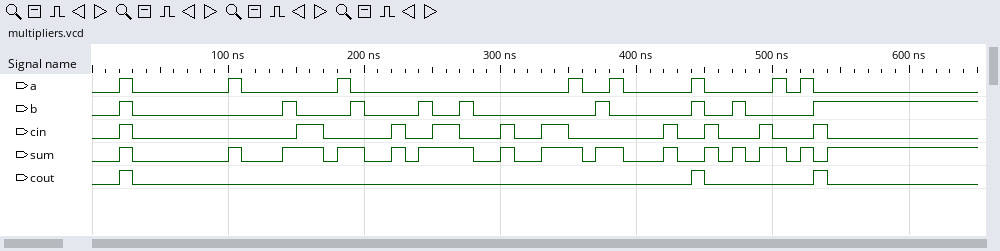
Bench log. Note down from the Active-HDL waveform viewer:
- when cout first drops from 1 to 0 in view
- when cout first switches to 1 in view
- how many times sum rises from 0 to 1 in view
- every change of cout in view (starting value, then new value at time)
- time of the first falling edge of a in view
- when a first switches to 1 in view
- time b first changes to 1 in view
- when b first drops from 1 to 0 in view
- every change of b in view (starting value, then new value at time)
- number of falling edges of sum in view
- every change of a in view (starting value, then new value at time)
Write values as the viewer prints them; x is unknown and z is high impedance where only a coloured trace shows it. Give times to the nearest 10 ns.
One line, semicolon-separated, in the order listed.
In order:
30 ns; 20 ns; 15; 0, 1 at 20 ns, 0 at 30 ns, 1 at 440 ns, 0 at 450 ns, 1 at 530 ns, 0 at 540 ns; 30 ns; 20 ns; 20 ns; 30 ns; 0, 1 at 20 ns, 0 at 30 ns, 1 at 140 ns, 0 at 150 ns, 1 at 190 ns, 0 at 200 ns, 1 at 240 ns, 0 at 250 ns, 1 at 270 ns, 0 at 280 ns, 1 at 370 ns, 0 at 380 ns, 1 at 440 ns, 0 at 450 ns, 1 at 470 ns, 0 at 480 ns, 1 at 530 ns; 14; 0, 1 at 20 ns, 0 at 30 ns, 1 at 100 ns, 0 at 110 ns, 1 at 180 ns, 0 at 190 ns, 1 at 350 ns, 0 at 360 ns, 1 at 380 ns, 0 at 390 ns, 1 at 440 ns, 0 at 450 ns, 1 at 500 ns, 0 at 510 ns, 1 at 520 ns, 0 at 530 ns
